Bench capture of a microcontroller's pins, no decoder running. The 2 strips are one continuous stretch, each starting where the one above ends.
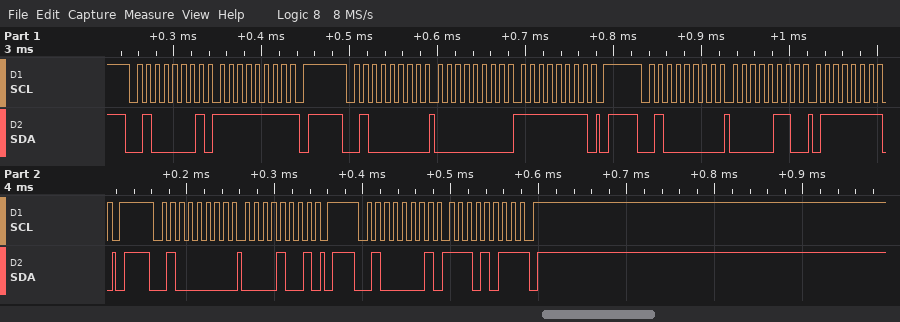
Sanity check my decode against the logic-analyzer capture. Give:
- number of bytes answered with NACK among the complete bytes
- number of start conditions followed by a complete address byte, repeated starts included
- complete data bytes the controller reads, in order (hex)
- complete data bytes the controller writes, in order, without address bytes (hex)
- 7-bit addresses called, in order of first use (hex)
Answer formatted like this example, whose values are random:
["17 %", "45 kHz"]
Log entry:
["2", "5", "FF EB", "00 FF 06 7F 09", "0x20"]
